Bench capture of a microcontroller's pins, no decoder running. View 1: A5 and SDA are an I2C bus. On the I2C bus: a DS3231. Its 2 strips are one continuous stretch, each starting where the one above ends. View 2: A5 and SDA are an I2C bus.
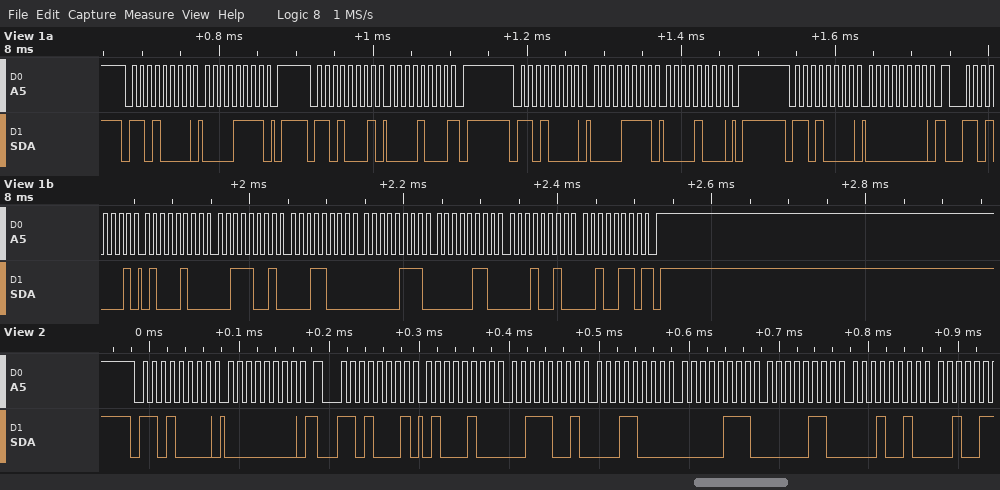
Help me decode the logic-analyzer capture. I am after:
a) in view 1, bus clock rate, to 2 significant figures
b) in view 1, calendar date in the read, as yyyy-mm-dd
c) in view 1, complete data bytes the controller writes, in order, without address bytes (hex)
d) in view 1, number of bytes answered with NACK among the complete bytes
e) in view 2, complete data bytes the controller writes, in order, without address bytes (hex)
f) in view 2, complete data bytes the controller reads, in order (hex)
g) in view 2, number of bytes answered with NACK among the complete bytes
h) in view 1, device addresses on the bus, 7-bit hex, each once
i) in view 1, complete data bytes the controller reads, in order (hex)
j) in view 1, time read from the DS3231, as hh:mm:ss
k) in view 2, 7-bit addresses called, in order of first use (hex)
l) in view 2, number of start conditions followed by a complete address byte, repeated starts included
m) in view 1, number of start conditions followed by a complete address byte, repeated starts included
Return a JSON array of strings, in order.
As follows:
["100 kHz", "2026-12-06", "0F 0F 08 00", "2", "00", "44 39 18 07 06 12", "0", "0x68", "08 44 39 18 07 06 12 26", "18:39:44", "0x68", "2", "5"]
